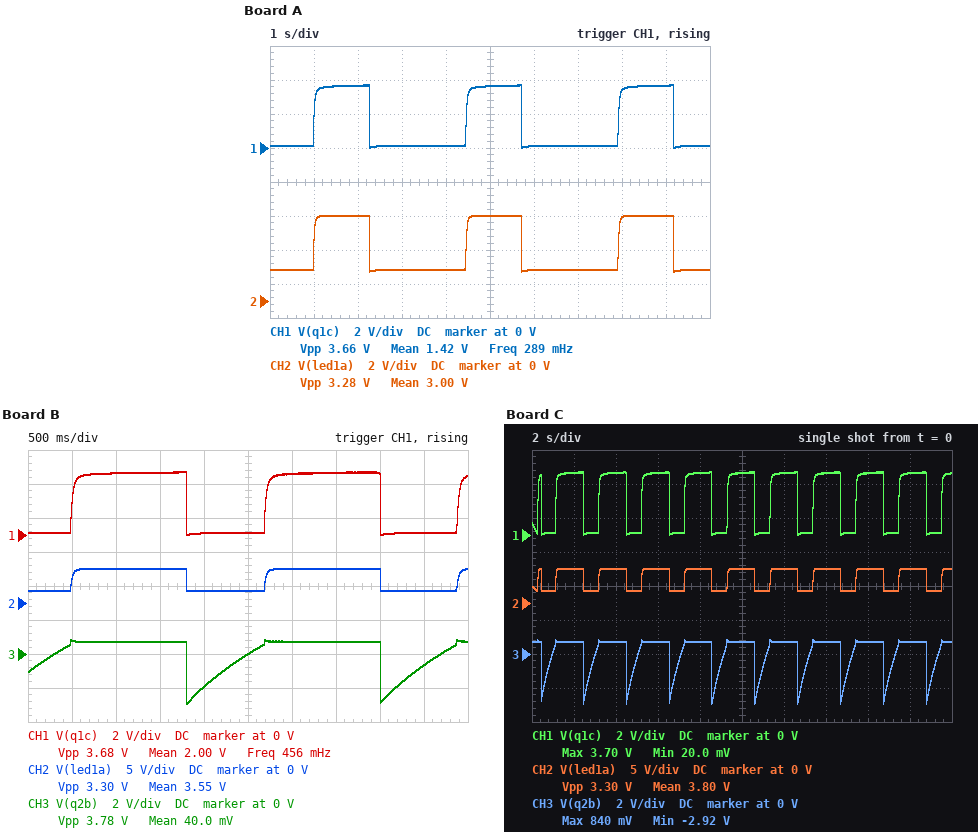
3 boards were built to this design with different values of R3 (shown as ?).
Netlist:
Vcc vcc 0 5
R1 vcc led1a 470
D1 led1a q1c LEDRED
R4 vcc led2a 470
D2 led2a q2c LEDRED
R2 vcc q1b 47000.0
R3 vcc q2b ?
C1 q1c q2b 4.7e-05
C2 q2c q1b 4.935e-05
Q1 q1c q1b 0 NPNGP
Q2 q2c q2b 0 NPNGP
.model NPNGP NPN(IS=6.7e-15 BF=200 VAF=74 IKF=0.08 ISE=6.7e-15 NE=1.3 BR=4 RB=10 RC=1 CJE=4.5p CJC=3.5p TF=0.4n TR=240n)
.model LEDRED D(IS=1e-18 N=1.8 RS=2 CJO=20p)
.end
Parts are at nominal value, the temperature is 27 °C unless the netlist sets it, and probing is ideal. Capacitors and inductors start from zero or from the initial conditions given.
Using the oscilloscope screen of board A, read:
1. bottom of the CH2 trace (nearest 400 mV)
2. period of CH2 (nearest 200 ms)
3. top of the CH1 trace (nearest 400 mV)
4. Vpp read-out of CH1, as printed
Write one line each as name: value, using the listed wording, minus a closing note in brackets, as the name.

bottom of the CH2 trace: 1.6 V
period of CH2: 3.4 s
top of the CH1 trace: 3.6 V
Vpp read-out of CH1, as printed: 3.66 V
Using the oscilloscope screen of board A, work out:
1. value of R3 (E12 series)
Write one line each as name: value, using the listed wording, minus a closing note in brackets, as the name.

value of R3: 82 kΩ
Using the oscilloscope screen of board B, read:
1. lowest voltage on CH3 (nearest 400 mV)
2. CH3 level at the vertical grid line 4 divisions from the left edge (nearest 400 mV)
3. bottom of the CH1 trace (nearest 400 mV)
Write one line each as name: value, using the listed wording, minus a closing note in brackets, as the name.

lowest voltage on CH3: -2.8 V
CH3 level at the vertical grid line 4 divisions from the left edge: -2.0 V
bottom of the CH1 trace: 0 V
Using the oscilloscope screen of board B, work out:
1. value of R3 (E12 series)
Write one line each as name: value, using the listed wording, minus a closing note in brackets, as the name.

value of R3: 33 kΩ
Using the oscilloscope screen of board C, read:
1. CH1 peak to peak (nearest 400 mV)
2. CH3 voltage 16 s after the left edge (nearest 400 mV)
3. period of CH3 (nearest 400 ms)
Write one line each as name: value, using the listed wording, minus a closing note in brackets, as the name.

CH1 peak to peak: 3.6 V
CH3 voltage 16 s after the left edge: 800 mV
period of CH3: 2.0 s
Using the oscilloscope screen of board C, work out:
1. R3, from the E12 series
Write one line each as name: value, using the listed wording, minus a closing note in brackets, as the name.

R3, from the E12 series: 27 kΩ
